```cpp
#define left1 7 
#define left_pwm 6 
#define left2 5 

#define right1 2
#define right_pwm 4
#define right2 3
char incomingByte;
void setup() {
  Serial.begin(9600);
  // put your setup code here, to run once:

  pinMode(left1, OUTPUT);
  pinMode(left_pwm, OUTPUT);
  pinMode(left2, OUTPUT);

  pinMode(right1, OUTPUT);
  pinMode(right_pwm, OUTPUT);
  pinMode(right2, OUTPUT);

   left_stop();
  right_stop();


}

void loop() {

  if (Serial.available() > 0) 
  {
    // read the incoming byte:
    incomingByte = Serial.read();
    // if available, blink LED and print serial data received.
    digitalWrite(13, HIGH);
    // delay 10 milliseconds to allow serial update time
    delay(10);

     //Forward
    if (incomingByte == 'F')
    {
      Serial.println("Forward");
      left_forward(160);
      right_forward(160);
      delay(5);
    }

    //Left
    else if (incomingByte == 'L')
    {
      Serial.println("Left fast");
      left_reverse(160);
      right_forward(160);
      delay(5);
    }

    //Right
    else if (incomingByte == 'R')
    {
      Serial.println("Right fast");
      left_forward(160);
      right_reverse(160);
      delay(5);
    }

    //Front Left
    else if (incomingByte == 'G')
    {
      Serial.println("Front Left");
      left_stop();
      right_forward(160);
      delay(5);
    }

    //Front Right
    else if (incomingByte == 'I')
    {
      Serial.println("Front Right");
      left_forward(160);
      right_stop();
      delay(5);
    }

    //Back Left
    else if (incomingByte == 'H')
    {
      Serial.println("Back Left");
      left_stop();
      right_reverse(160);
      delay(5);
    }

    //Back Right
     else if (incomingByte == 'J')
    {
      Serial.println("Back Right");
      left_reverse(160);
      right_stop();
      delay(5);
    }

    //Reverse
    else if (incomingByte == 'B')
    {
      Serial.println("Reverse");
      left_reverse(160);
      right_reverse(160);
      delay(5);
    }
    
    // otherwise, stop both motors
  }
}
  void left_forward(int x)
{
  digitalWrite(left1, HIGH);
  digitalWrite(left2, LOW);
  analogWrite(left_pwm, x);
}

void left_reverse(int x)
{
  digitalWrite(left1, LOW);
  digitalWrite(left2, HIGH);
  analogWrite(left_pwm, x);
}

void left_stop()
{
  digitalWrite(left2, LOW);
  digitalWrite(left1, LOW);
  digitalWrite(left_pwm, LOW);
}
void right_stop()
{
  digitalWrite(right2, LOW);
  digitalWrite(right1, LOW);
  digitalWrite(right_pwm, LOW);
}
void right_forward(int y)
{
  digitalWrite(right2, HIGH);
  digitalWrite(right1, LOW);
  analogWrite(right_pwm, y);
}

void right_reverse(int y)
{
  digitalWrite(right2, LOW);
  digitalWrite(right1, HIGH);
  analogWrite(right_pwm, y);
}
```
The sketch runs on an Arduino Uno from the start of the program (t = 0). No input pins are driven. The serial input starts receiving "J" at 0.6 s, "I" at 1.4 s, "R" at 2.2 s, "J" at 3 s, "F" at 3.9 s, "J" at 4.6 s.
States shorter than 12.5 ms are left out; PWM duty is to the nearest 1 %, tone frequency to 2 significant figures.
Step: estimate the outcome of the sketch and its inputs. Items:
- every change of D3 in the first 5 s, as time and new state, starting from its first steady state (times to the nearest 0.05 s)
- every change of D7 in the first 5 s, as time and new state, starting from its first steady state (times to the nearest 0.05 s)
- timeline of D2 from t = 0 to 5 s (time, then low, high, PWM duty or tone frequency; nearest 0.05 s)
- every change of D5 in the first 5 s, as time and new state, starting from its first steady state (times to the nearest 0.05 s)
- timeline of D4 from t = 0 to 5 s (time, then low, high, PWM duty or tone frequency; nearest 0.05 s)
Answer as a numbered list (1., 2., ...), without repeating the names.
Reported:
1. 0 s low; 3.9 s high; 4.6 s low
2. 0 s low; 1.4 s high; 3 s low; 3.9 s high; 4.6 s low
3. 0 s low; 2.2 s high; 3 s low
4. 0 s low; 0.6 s high; 1.4 s low; 3 s high; 3.9 s low; 4.6 s high
5. 0 s low; 2.2 s high; 3 s low; 3.9 s high; 4.6 s low
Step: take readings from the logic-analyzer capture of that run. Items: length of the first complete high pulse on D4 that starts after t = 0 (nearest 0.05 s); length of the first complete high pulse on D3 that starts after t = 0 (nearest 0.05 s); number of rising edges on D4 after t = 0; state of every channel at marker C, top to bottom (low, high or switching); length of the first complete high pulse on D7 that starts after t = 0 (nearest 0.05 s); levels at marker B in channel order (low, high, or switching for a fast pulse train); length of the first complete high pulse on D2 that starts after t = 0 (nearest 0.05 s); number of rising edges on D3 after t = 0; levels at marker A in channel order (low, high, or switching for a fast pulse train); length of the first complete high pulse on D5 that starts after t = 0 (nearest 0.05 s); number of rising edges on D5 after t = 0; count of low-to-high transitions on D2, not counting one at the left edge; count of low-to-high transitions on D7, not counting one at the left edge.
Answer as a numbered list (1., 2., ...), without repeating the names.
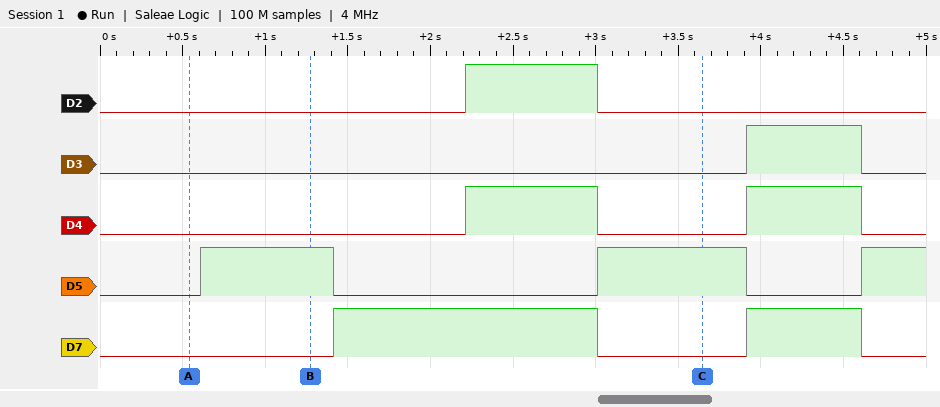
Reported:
1. 0.80 s
2. 0.70 s
3. 2
4. D2 low, D3 low, D4 low, D5 high, D7 low
5. 1.60 s
6. D2 low, D3 low, D4 low, D5 high, D7 low
7. 0.80 s
8. 1
9. D2 low, D3 low, D4 low, D5 low, D7 low
10. 0.80 s
11. 3
12. 1
13. 2
